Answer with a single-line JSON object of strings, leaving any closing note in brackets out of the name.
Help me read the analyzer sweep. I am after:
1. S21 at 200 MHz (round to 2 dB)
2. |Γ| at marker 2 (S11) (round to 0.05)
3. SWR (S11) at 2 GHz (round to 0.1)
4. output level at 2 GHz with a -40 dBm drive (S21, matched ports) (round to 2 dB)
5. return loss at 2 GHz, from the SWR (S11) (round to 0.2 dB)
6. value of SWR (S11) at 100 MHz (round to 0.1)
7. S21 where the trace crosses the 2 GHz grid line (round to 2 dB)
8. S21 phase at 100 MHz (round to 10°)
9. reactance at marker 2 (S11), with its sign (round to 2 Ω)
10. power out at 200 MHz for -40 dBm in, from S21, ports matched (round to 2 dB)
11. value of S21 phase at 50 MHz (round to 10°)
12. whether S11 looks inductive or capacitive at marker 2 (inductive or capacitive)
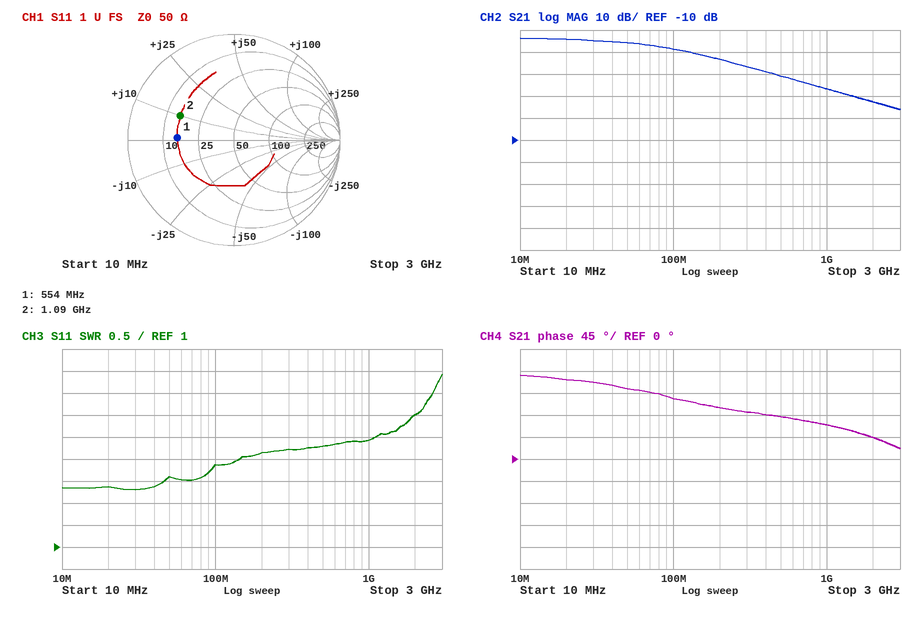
{"S21 at 200 MHz": "26 dB", "|Γ| at marker 2 (S11)": "0.55", "SWR (S11) at 2 GHz": "4.0", "output level at 2 GHz with a -40 dBm drive (S21, matched ports)": "-32 dBm", "return loss at 2 GHz, from the SWR (S11)": "4.4 dB", "value of SWR (S11) at 100 MHz": "2.9", "S21 where the trace crosses the 2 GHz grid line": "8 dB", "S21 phase at 100 MHz": "120°", "reactance at marker 2 (S11), with its sign": "+10 Ω", "power out at 200 MHz for -40 dBm in, from S21, ports matched": "-14 dBm", "value of S21 phase at 50 MHz": "140°", "whether S11 looks inductive or capacitive at marker 2": "inductive"}
